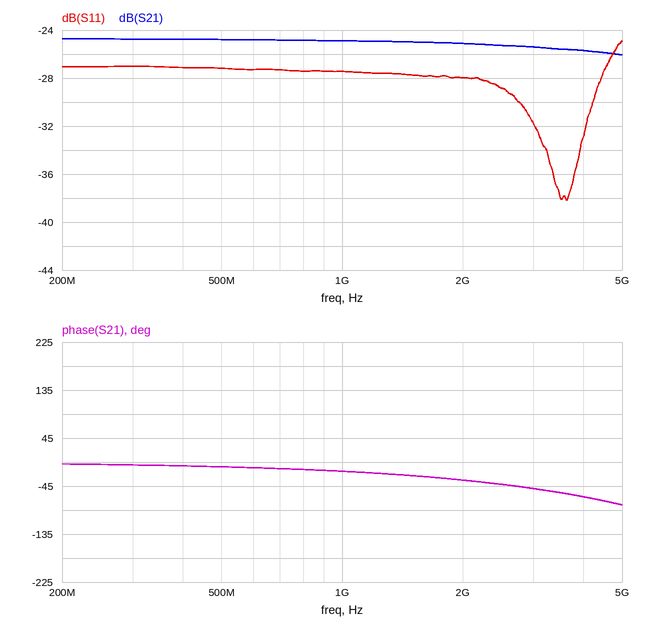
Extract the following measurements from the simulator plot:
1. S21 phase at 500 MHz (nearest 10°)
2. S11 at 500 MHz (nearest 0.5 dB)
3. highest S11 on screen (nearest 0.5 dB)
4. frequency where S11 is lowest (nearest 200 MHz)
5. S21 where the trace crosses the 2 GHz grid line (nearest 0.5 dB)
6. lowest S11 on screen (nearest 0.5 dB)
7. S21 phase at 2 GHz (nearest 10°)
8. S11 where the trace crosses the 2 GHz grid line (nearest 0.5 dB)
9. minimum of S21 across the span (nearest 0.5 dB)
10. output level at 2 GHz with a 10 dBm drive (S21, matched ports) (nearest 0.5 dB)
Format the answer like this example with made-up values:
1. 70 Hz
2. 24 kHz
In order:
1. -10°
2. -27.0 dB
3. -25.0 dB
4. 3.6 GHz
5. -25.0 dB
6. -38.0 dB
7. -30°
8. -28.0 dB
9. -26.0 dB
10. -15.0 dBm
